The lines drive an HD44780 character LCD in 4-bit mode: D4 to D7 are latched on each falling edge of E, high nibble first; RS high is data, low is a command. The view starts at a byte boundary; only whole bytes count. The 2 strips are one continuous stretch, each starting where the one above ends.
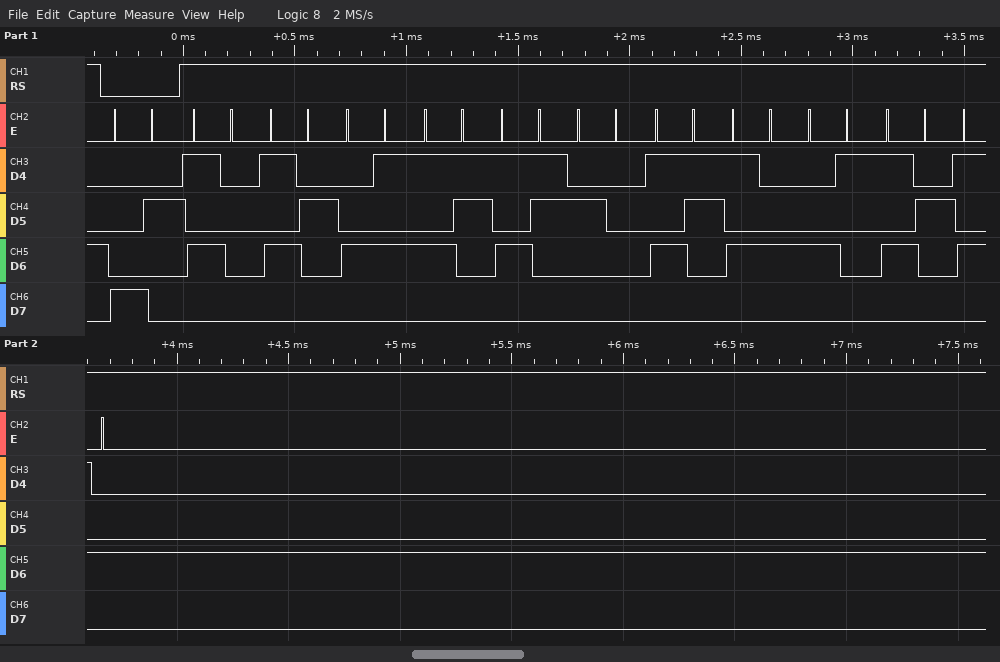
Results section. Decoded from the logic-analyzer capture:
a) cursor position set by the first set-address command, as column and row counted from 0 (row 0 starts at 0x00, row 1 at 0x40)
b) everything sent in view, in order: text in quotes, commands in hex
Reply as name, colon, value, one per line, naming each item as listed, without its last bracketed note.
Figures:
cursor position set by the first set-address command, as column and row counted from 0: column 2, row 0
everything sent in view, in order: text in quotes, commands in hex: 0x82 "PRESS START"
